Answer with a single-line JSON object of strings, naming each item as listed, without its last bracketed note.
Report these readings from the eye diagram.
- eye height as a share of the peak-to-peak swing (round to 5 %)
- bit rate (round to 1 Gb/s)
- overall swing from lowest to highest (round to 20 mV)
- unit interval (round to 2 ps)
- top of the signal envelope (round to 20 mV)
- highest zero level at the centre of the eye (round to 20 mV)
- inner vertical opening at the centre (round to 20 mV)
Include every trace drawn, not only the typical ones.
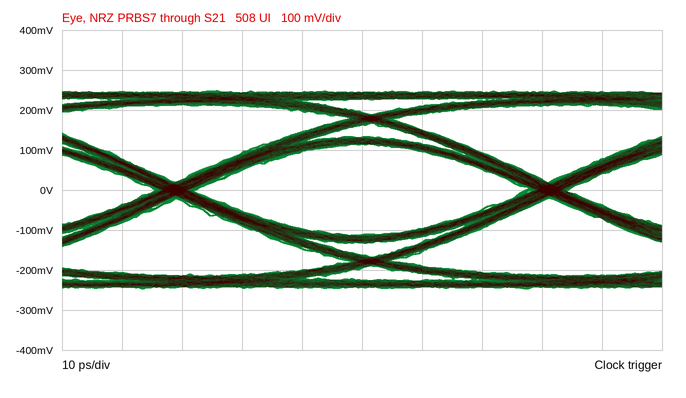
{"eye height as a share of the peak-to-peak swing": "45 %", "bit rate": "16 Gb/s", "overall swing from lowest to highest": "500 mV", "unit interval": "62 ps", "top of the signal envelope": "240 mV", "highest zero level at the centre of the eye": "-120 mV", "inner vertical opening at the centre": "220 mV"}
